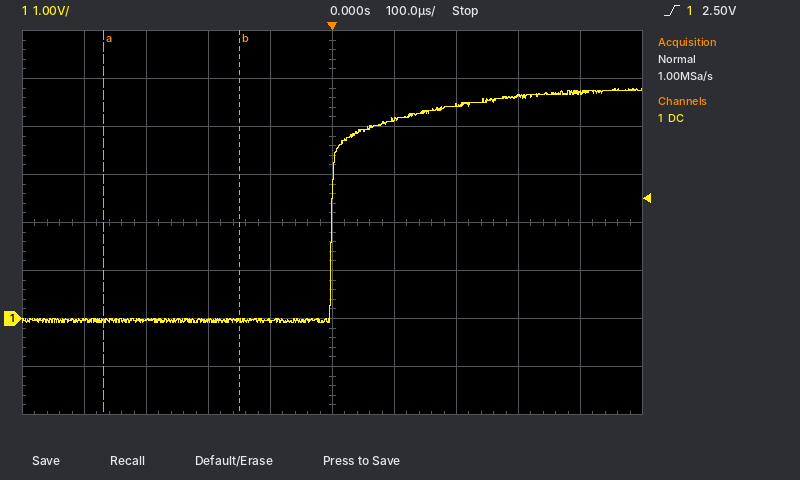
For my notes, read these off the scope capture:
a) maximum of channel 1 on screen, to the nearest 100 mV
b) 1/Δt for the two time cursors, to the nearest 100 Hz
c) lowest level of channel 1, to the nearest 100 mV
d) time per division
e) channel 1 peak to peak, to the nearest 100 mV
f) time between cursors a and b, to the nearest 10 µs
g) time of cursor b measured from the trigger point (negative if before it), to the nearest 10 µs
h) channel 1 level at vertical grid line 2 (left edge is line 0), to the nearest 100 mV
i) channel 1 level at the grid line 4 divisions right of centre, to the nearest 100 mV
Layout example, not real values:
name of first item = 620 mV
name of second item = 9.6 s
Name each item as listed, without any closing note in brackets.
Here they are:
maximum of channel 1 on screen, to the nearest 100 mV = 4.8 V
1/Δt for the two time cursors, to the nearest 100 Hz = 4.5 kHz
lowest level of channel 1, to the nearest 100 mV = -100 mV
time per division = 100 µs
channel 1 peak to peak, to the nearest 100 mV = 4.9 V
time between cursors a and b, to the nearest 10 µs = 220 µs
time of cursor b measured from the trigger point (negative if before it), to the nearest 10 µs = -150 µs
channel 1 level at vertical grid line 2 (left edge is line 0), to the nearest 100 mV = 0.0 V
channel 1 level at the grid line 4 divisions right of centre, to the nearest 100 mV = 4.7 V
